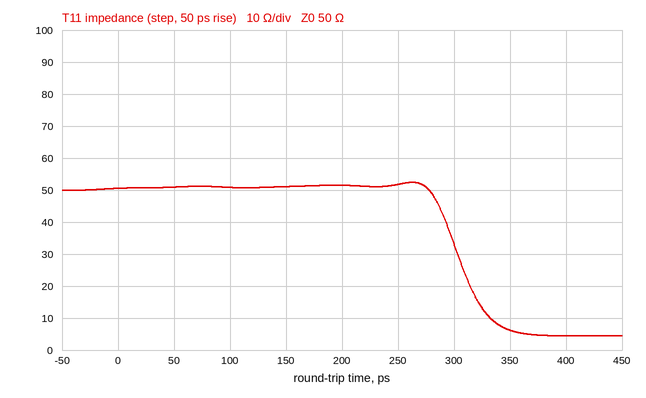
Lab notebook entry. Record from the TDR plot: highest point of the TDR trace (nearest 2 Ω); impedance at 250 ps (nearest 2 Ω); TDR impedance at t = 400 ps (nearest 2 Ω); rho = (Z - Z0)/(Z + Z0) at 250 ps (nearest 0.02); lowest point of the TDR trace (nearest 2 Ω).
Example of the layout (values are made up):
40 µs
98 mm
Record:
52 Ω
52 Ω
4 Ω
+0.02
4 Ω
